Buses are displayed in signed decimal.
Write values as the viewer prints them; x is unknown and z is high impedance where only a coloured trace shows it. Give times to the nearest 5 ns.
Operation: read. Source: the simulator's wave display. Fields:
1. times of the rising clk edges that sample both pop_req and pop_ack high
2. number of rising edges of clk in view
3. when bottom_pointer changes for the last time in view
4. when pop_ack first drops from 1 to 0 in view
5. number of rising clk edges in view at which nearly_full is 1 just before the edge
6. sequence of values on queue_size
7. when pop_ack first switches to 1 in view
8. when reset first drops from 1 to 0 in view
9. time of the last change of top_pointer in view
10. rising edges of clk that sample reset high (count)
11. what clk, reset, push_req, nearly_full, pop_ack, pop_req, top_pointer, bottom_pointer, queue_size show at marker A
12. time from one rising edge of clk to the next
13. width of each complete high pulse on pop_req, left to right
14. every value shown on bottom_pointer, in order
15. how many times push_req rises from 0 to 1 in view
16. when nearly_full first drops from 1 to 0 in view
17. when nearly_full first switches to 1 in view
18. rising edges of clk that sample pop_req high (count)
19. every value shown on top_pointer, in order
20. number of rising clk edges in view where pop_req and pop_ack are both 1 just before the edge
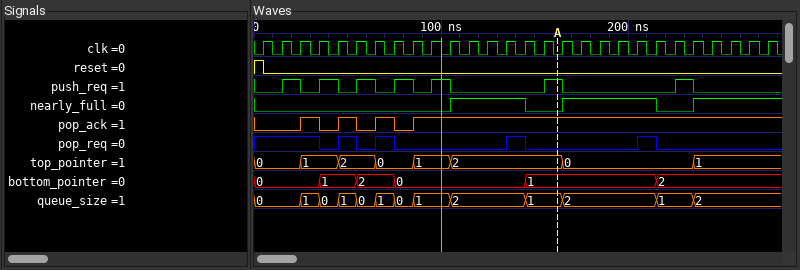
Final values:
35 ns, 55 ns, 75 ns, 145 ns, 215 ns
28
215 ns
35 ns
13
0, 1, 0, 1, 0, 1, 0, 1, 2, 1, 2, 1, 2
25 ns
5 ns
235 ns
1
clk=0, reset=0, push_req=1, nearly_full=0, pop_ack=1, pop_req=0, top_pointer=2, bottom_pointer=1, queue_size=1
10 ns
10 ns, 10 ns, 10 ns, 10 ns
0, 1, 2, 0, 1, 2
7
145 ns
105 ns
8
0, 1, 2, 0, 1, 2, 0, 1
5
